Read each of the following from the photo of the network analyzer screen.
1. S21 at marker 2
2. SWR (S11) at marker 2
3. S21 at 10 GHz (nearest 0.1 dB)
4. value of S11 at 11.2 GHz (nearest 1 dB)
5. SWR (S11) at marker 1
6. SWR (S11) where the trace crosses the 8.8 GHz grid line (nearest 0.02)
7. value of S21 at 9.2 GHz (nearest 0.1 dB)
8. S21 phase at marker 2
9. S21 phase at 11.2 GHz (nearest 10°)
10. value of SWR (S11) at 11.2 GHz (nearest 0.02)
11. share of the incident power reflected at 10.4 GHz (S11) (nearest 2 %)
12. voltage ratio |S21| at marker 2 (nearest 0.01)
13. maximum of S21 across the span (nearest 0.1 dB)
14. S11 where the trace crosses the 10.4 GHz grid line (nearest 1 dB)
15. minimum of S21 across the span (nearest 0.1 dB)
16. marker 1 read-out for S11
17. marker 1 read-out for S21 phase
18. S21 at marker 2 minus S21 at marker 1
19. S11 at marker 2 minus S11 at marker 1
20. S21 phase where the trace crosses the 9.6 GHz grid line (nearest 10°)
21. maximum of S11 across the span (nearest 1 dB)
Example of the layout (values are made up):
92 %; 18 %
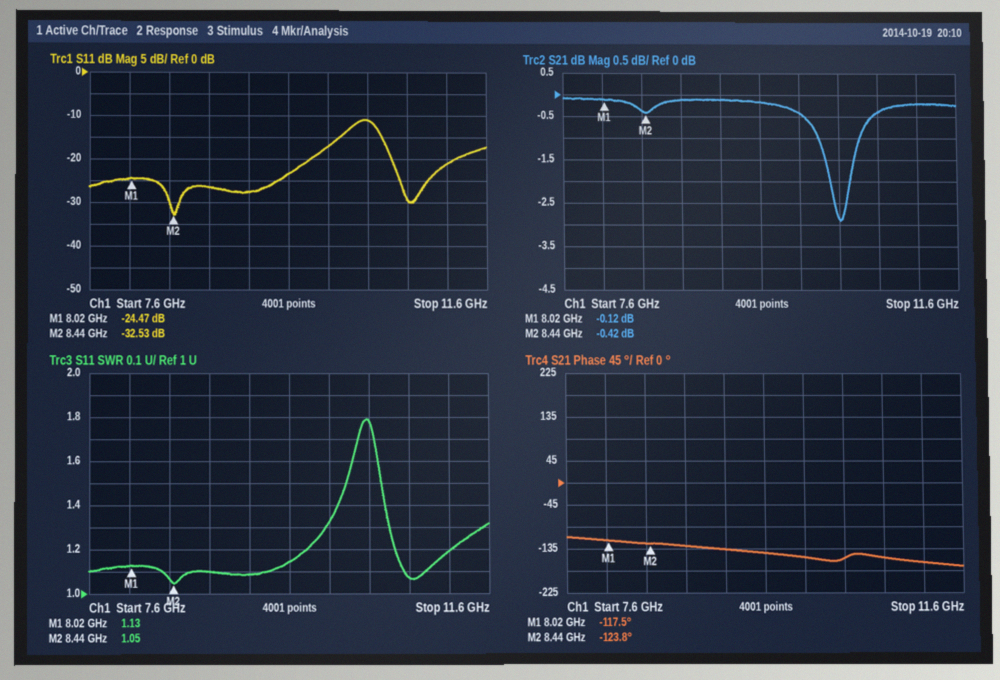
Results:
-0.42 dB; 1.05; -0.4 dB; -21 dB; 1.13; 1.10; -0.1 dB; -123.8°; -160°; 1.20; 8 %; 0.95; -0.1 dB; -11 dB; -2.9 dB; -24.47 dB; -117.5°; -0.30 dB; -8.06 dB; -140°; -11 dB
